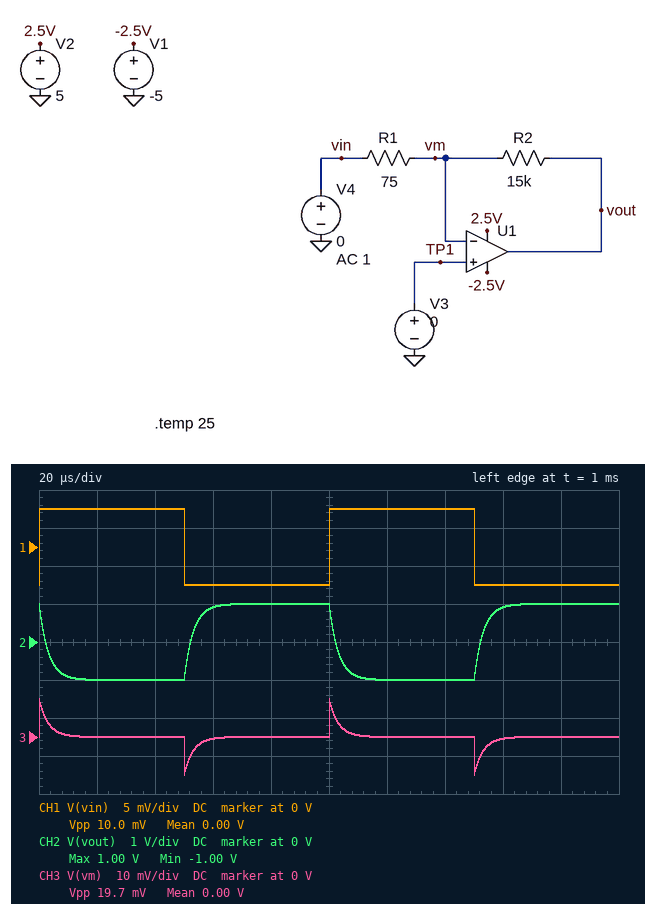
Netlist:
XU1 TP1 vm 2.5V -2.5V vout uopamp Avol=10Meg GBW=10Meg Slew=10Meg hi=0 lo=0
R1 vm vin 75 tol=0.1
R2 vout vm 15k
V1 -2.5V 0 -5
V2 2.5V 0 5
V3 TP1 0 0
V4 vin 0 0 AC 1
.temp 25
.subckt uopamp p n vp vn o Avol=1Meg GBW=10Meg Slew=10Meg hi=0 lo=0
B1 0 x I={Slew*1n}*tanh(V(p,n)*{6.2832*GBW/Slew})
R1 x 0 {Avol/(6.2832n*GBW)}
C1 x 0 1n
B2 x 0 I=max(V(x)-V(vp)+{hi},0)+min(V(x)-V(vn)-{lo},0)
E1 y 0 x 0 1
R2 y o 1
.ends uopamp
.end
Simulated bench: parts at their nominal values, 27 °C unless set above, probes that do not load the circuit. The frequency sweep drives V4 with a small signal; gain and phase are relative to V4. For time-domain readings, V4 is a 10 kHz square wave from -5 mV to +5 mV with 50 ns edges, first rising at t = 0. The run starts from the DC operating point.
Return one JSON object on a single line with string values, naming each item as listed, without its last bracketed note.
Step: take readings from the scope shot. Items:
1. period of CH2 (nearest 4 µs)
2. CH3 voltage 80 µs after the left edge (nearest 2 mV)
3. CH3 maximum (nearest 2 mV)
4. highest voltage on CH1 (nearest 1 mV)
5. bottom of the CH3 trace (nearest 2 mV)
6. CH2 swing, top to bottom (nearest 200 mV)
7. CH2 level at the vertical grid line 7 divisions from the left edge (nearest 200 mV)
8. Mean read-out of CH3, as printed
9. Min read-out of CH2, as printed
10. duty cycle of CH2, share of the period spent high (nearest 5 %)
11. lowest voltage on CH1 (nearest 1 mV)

{"period of CH2": "100 µs", "CH3 voltage 80 µs after the left edge": "0 V", "CH3 maximum": "10 mV", "highest voltage on CH1": "5 mV", "bottom of the CH3 trace": "-10 mV", "CH2 swing, top to bottom": "2.0 V", "CH2 level at the vertical grid line 7 divisions from the left edge": "-1.0 V", "Mean read-out of CH3, as printed": "0.00 V", "Min read-out of CH2, as printed": "-1.00 V", "duty cycle of CH2, share of the period spent high": "50 %", "lowest voltage on CH1": "-5 mV"}
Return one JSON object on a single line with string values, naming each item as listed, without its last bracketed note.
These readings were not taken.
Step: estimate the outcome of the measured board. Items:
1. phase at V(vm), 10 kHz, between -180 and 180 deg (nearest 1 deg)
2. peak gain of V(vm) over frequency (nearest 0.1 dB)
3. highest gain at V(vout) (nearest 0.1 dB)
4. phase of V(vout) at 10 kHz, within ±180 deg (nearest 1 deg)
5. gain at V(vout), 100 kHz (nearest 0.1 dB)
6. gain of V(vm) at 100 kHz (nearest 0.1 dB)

{"phase at V(vm), 10 kHz, between -180 and 180 deg": "79 deg", "peak gain of V(vm) over frequency": "0 dB", "highest gain at V(vout)": "46.0 dB", "phase of V(vout) at 10 kHz, within ±180 deg": "169 deg", "gain at V(vout), 100 kHz": "39.0 dB", "gain of V(vm) at 100 kHz": "-1.0 dB"}
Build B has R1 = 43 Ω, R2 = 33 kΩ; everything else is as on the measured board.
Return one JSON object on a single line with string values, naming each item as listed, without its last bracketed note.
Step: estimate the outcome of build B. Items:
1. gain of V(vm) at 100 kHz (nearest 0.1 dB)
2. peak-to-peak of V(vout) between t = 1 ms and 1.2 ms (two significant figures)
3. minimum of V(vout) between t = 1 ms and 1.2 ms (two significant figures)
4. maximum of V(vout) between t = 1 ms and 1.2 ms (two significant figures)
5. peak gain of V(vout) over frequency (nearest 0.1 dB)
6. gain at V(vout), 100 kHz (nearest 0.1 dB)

{"gain of V(vm) at 100 kHz": "-0.1 dB", "peak-to-peak of V(vout) between t = 1 ms and 1.2 ms": "7.4 V", "minimum of V(vout) between t = 1 ms and 1.2 ms": "-3.7 V", "maximum of V(vout) between t = 1 ms and 1.2 ms": "3.7 V", "peak gain of V(vout) over frequency": "57.7 dB", "gain at V(vout), 100 kHz": "39.9 dB"}
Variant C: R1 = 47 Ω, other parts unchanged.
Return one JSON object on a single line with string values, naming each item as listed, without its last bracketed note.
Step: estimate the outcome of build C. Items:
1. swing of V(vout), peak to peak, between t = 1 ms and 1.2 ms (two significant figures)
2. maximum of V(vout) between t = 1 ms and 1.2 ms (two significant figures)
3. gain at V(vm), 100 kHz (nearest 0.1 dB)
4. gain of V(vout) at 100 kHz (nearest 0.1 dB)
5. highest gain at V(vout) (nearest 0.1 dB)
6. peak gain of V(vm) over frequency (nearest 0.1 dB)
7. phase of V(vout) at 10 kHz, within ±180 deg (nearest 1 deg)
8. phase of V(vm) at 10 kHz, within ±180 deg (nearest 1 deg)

{"swing of V(vout), peak to peak, between t = 1 ms and 1.2 ms": "3.2 V", "maximum of V(vout) between t = 1 ms and 1.2 ms": "1.6 V", "gain at V(vm), 100 kHz": "-0.4 dB", "gain of V(vout) at 100 kHz": "39.6 dB", "highest gain at V(vout)": "50.1 dB", "peak gain of V(vm) over frequency": "0 dB", "phase of V(vout) at 10 kHz, within ±180 deg": "162 deg", "phase of V(vm) at 10 kHz, within ±180 deg": "72 deg"}
